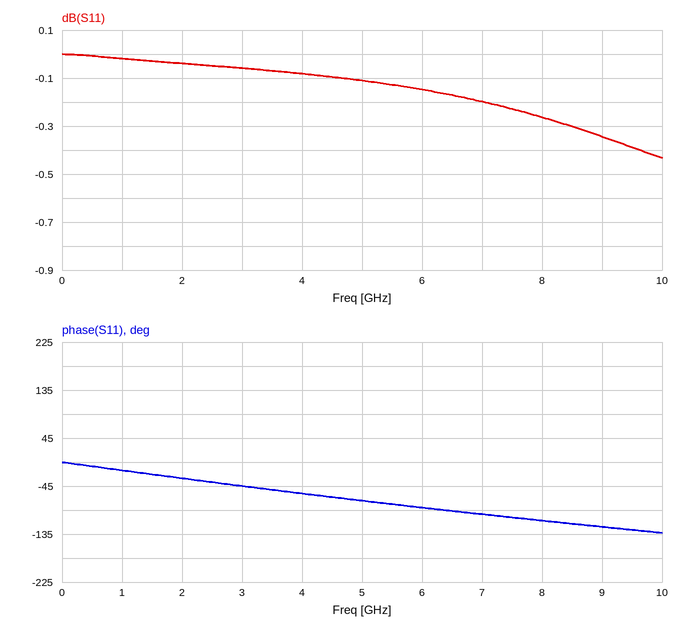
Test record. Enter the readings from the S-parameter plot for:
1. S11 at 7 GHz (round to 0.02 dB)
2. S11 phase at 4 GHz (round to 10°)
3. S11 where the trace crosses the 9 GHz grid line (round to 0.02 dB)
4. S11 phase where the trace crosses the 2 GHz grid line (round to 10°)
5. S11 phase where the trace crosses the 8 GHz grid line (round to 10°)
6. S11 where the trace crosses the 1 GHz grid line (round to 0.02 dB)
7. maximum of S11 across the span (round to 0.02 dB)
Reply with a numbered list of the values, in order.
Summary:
1. -0.20 dB
2. -60°
3. -0.34 dB
4. -30°
5. -110°
6. -0.02 dB
7. 0.00 dB
